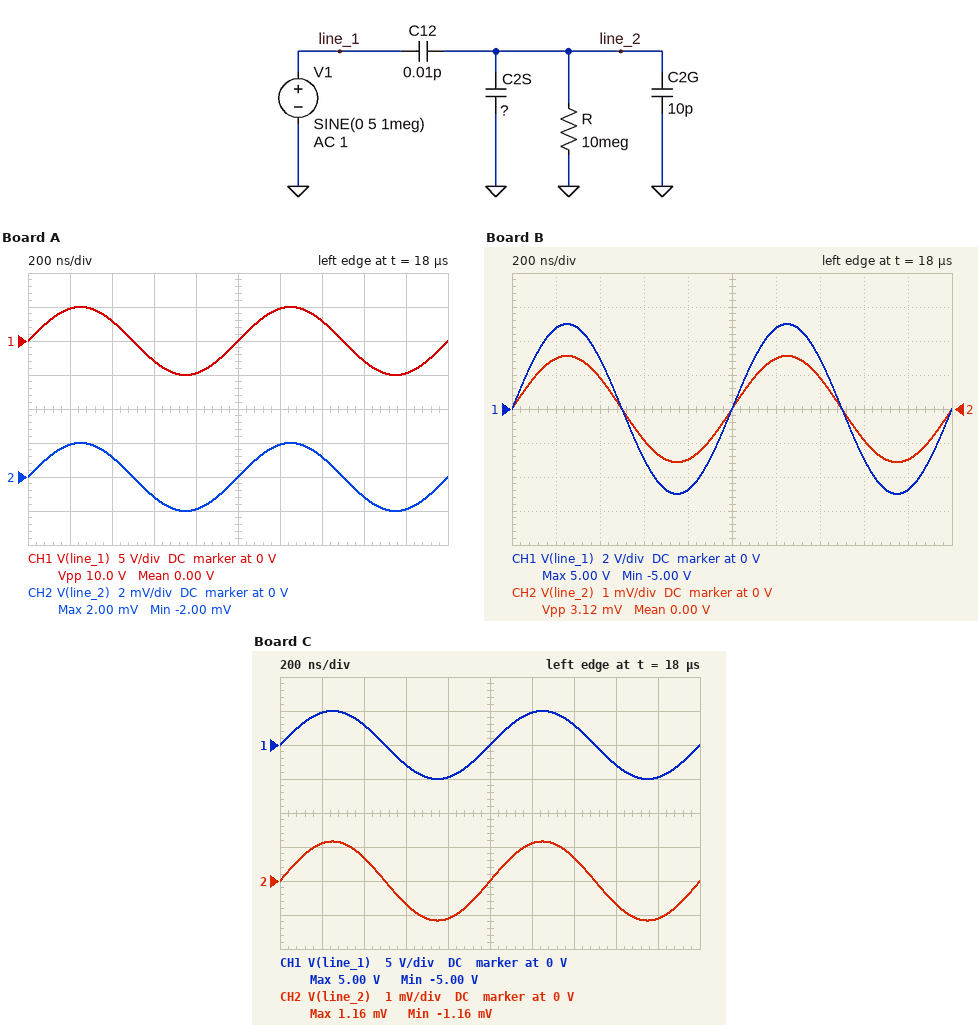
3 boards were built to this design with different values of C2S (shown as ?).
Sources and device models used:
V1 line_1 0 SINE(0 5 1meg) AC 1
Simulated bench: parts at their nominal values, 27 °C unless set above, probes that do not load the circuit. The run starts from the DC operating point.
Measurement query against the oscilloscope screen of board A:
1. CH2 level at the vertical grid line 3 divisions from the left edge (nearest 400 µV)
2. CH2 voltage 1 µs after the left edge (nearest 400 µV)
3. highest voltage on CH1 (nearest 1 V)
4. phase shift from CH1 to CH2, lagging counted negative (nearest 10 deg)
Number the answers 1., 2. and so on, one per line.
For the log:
1. -1.2 mV
2. 0 V
3. 5 V
4. 0 deg
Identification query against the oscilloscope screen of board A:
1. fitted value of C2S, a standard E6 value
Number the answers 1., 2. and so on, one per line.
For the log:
1. 15 pF
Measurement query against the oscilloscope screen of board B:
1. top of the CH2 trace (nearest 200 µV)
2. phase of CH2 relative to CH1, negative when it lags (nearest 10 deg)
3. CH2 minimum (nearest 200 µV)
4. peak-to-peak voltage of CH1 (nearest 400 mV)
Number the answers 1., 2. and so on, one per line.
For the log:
1. 1.6 mV
2. 0 deg
3. -1.6 mV
4. 10.0 V
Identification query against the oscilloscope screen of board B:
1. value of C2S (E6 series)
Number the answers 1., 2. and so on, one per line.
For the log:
1. 22 pF
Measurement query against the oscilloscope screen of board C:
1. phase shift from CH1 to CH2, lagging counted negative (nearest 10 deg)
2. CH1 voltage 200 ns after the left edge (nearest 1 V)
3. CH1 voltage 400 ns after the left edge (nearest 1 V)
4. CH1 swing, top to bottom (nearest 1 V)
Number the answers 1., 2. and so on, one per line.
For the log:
1. 0 deg
2. 5 V
3. 3 V
4. 10 V
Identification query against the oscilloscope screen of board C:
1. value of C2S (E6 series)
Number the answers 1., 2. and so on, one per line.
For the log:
1. 33 pF
